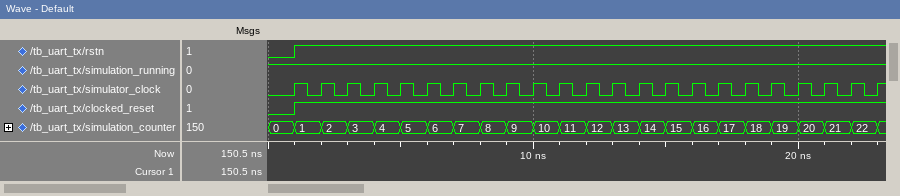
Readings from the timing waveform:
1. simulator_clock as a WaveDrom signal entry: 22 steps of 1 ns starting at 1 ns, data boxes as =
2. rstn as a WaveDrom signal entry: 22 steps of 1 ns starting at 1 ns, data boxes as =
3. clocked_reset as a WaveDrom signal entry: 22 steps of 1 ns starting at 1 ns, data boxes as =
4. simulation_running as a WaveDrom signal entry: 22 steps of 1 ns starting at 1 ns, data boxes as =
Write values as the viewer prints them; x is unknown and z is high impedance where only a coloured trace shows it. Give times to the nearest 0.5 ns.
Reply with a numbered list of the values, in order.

1. {name: 'simulator_clock', wave: 'p.....................'}
2. {name: 'rstn', wave: '1.....................'}
3. {name: 'clocked_reset', wave: '1.....................'}
4. {name: 'simulation_running', wave: '1.....................'}
